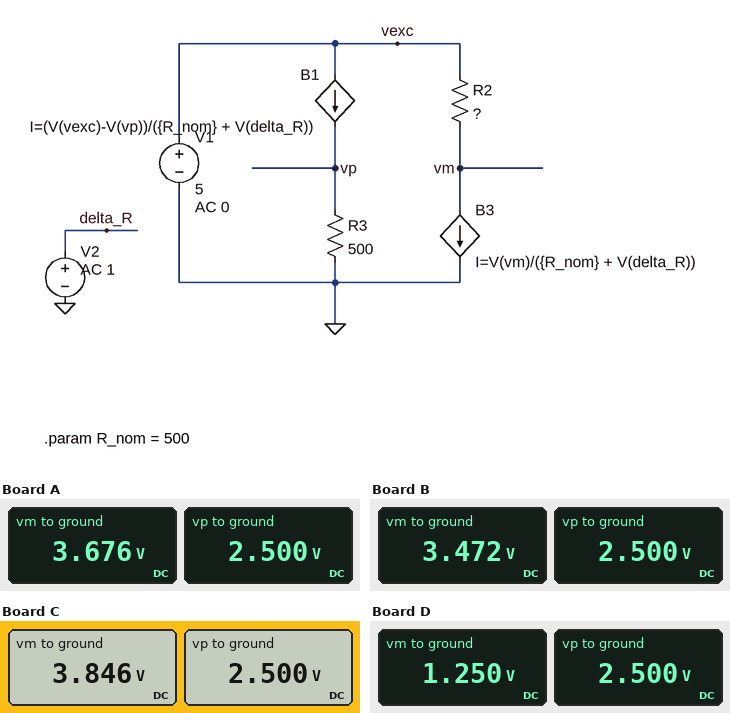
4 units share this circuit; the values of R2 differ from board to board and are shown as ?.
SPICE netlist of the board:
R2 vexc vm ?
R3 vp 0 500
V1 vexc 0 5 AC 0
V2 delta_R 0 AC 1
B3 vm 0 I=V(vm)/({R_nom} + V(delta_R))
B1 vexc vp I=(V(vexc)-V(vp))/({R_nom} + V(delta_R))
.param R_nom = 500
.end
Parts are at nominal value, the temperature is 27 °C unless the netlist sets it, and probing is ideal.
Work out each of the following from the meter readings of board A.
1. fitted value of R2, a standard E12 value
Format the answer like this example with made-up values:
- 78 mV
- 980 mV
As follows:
- 180 Ω
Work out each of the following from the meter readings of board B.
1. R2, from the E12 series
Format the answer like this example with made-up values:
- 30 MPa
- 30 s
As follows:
- 220 Ω
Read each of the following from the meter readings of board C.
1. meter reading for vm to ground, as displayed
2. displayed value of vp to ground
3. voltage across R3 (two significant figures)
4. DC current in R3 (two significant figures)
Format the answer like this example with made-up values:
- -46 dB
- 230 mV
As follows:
- 3.846 V
- 2.500 V
- 2.5 V
- 5.0 mA
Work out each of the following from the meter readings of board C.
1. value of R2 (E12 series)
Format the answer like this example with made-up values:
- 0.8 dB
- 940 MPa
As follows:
- 150 Ω
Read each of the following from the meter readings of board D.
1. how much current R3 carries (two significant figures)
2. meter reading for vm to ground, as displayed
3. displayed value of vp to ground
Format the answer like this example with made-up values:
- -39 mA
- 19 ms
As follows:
- 5.0 mA
- 1.250 V
- 2.500 V
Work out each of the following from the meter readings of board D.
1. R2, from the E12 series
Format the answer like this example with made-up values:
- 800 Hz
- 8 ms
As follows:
- 1.5 kΩ
